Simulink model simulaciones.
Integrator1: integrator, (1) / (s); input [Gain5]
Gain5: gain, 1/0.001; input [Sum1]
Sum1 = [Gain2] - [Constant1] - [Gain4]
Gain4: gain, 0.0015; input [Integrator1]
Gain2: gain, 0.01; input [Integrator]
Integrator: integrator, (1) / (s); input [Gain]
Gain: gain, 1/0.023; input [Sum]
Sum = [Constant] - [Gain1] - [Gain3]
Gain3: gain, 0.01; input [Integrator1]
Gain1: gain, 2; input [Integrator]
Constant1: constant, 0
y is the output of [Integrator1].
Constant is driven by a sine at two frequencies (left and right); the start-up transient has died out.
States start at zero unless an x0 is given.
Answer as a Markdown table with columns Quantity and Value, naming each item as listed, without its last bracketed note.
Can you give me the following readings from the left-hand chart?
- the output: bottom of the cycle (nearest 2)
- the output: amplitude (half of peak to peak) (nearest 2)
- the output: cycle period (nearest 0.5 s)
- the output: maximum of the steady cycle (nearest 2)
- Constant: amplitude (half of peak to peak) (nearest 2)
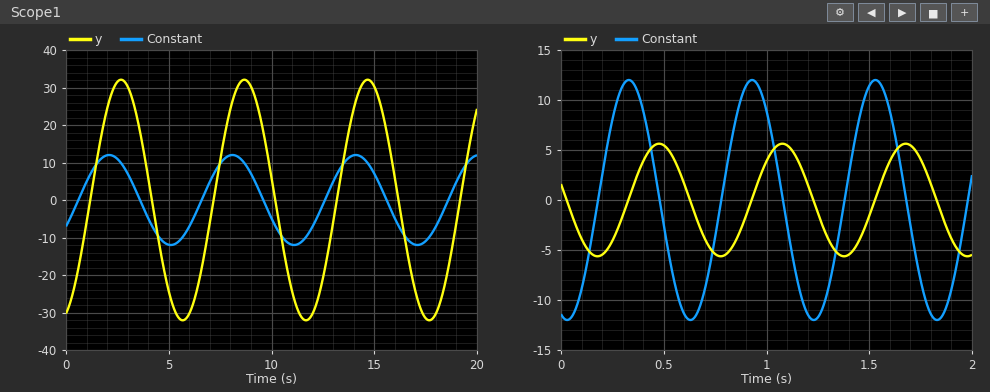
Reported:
| Quantity | Value |
|---|---|
| the output: bottom of the cycle | -32 |
| the output: amplitude (half of peak to peak) | 32 |
| the output: cycle period | 6.0 s |
| the output: maximum of the steady cycle | 32 |
| Constant: amplitude (half of peak to peak) | 12 |
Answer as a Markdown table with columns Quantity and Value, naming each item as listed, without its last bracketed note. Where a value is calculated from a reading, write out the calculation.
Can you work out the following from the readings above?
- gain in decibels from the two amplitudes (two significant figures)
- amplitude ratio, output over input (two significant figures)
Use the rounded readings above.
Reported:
| Quantity | Value |
|---|---|
| gain in decibels from the two amplitudes | 20 log10(32 / 12) = 8.5 dB |
| amplitude ratio, output over input | 32 / 12 = 2.7 |
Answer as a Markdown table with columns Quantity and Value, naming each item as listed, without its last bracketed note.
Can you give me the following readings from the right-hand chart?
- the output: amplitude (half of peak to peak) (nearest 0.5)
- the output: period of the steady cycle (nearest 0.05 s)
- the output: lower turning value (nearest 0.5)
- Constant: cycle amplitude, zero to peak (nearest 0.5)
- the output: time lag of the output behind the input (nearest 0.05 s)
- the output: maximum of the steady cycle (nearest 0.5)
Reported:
| Quantity | Value |
|---|---|
| the output: amplitude (half of peak to peak) | 5.5 |
| the output: period of the steady cycle | 0.60 s |
| the output: lower turning value | -5.5 |
| Constant: cycle amplitude, zero to peak | 12.0 |
| the output: time lag of the output behind the input | 0.15 s |
| the output: maximum of the steady cycle | 5.5 |
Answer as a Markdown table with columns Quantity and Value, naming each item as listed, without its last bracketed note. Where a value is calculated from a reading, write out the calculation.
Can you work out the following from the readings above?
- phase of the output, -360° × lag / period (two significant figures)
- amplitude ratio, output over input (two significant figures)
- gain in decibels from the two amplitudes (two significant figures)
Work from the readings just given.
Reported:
| Quantity | Value |
|---|---|
| phase of the output, -360° × lag / period | -360 × 0.15 / 0.6 = -90° |
| amplitude ratio, output over input | 5.5 / 12 = 0.46 |
| gain in decibels from the two amplitudes | 20 log10(5.5 / 12) = -6.8 dB |
